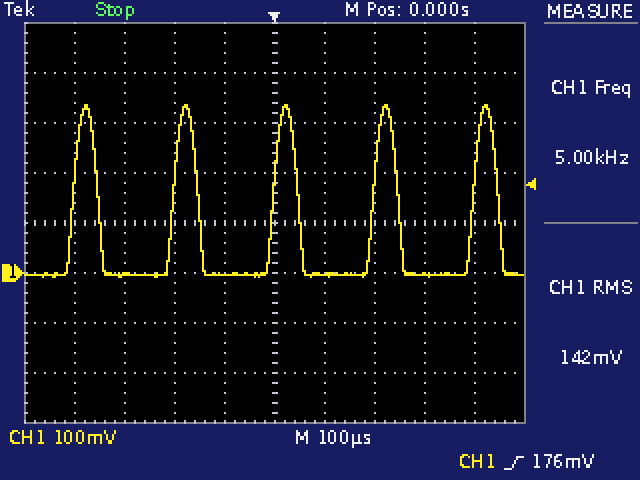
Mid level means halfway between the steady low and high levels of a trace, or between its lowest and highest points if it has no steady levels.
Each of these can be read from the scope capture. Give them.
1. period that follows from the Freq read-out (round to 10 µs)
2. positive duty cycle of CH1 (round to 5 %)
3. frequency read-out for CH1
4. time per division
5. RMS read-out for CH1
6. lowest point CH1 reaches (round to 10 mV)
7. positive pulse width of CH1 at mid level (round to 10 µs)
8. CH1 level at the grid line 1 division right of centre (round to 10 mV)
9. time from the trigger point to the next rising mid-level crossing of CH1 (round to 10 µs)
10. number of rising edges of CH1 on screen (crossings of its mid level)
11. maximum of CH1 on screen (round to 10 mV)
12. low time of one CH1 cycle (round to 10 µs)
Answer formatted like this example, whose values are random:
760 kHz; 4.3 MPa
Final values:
200 µs; 25 %; 5.00 kHz; 100 µs; 142 mV; -10 mV; 50 µs; 0 mV; 200 µs; 5; 340 mV; 150 µs
